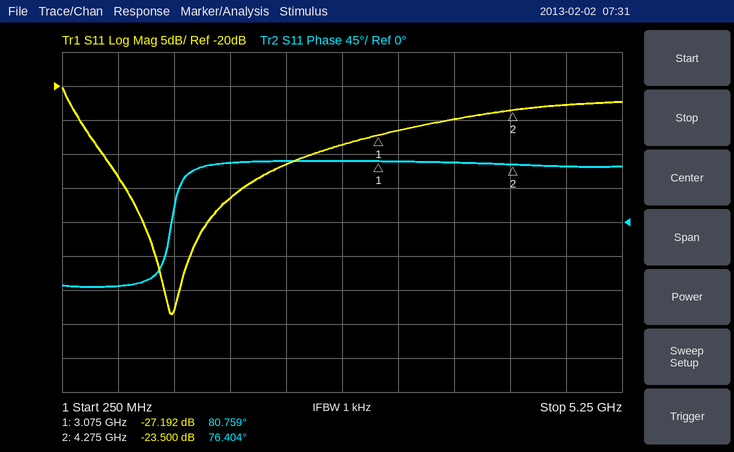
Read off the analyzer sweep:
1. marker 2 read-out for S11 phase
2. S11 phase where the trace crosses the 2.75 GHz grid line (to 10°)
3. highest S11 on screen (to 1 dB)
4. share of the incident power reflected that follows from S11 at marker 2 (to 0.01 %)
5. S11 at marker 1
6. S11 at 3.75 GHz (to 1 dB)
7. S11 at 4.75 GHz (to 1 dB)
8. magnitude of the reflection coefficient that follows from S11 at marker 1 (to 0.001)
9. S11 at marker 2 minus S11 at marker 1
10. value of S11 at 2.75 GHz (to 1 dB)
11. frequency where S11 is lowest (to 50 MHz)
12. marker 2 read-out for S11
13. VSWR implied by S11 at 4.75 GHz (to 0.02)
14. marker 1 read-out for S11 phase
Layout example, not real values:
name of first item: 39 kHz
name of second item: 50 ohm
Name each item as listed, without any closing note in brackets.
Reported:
marker 2 read-out for S11 phase: 76.404°
S11 phase where the trace crosses the 2.75 GHz grid line: 80°
highest S11 on screen: -20 dB
share of the incident power reflected that follows from S11 at marker 2: 0.45 %
S11 at marker 1: -27.192 dB
S11 at 3.75 GHz: -25 dB
S11 at 4.75 GHz: -23 dB
magnitude of the reflection coefficient that follows from S11 at marker 1: 0.044
S11 at marker 2 minus S11 at marker 1: 3.692 dB
value of S11 at 2.75 GHz: -29 dB
frequency where S11 is lowest: 1.25 GHz
marker 2 read-out for S11: -23.500 dB
VSWR implied by S11 at 4.75 GHz: 1.16
marker 1 read-out for S11 phase: 80.759°
